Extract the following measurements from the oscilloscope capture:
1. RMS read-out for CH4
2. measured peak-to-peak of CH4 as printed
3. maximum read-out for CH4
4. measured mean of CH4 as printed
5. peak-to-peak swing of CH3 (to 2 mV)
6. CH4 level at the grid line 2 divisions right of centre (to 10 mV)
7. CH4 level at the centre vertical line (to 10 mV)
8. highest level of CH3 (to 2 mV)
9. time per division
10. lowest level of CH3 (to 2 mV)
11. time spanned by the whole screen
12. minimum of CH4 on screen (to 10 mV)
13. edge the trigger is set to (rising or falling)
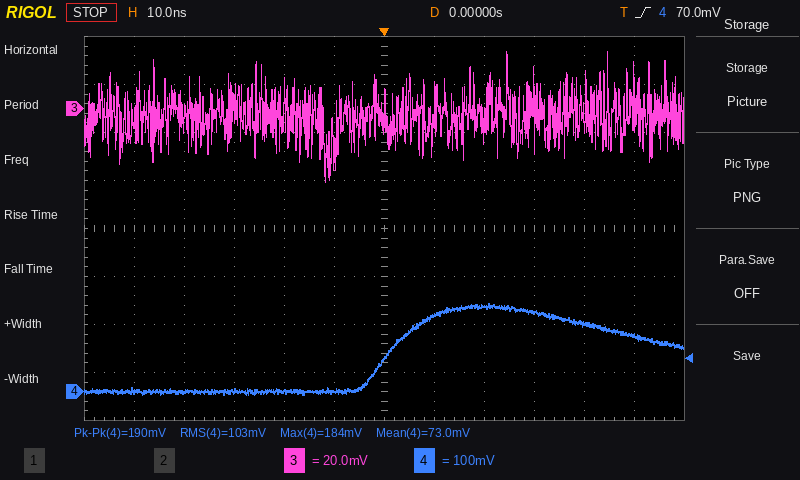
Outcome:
103 mV
190 mV
184 mV
73.0 mV
54 mV
180 mV
70 mV
24 mV
10 ns
-30 mV
120 ns
-10 mV
rising
